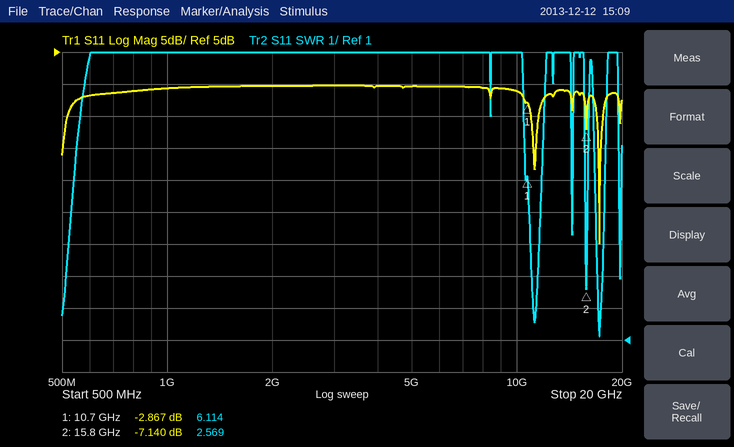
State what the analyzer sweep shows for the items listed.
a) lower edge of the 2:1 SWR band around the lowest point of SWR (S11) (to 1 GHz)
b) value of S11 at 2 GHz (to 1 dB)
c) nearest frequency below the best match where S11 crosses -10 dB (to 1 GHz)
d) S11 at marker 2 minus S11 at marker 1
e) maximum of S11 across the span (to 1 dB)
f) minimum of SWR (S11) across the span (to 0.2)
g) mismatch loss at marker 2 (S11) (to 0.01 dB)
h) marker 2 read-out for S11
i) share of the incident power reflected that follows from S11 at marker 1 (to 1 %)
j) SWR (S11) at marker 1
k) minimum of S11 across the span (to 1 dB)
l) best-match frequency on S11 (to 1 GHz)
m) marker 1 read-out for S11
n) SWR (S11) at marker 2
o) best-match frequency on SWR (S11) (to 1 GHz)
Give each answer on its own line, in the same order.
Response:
17 GHz
0 dB
17 GHz
-4.273 dB
0 dB
1.2
0.93 dB
-7.140 dB
52 %
6.114
-25 dB
17 GHz
-2.867 dB
2.569
17 GHz
